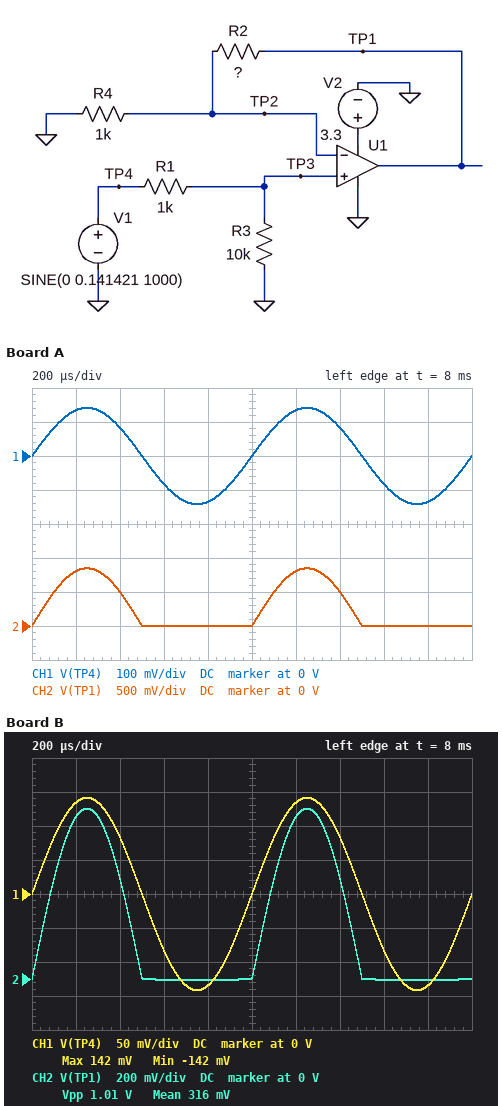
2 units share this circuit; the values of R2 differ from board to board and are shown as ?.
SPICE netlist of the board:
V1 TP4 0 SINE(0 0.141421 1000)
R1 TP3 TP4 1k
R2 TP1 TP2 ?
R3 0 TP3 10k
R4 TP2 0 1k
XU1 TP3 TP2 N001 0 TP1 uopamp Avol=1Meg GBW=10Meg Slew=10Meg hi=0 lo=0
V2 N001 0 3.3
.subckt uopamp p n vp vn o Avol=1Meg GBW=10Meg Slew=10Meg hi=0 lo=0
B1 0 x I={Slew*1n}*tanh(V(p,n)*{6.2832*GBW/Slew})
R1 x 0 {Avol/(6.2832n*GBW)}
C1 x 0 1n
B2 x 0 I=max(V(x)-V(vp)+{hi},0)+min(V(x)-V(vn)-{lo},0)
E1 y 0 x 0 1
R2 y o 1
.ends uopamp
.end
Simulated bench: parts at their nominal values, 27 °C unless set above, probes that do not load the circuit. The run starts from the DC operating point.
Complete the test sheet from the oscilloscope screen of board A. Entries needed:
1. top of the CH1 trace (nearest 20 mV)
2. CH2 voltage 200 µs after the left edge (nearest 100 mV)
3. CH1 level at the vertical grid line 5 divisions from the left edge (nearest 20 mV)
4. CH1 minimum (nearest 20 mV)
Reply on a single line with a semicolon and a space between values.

140 mV; 800 mV; 0 V; -140 mV
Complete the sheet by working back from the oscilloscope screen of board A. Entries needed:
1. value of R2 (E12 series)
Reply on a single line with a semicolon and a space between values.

5.6 kΩ
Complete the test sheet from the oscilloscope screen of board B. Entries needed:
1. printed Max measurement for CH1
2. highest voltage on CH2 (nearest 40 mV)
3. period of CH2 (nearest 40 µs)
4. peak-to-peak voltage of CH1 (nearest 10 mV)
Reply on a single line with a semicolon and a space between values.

142 mV; 1.00 V; 1.00 ms; 280 mV
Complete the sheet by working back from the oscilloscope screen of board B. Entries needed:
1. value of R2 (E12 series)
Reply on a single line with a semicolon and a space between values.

6.8 kΩ
